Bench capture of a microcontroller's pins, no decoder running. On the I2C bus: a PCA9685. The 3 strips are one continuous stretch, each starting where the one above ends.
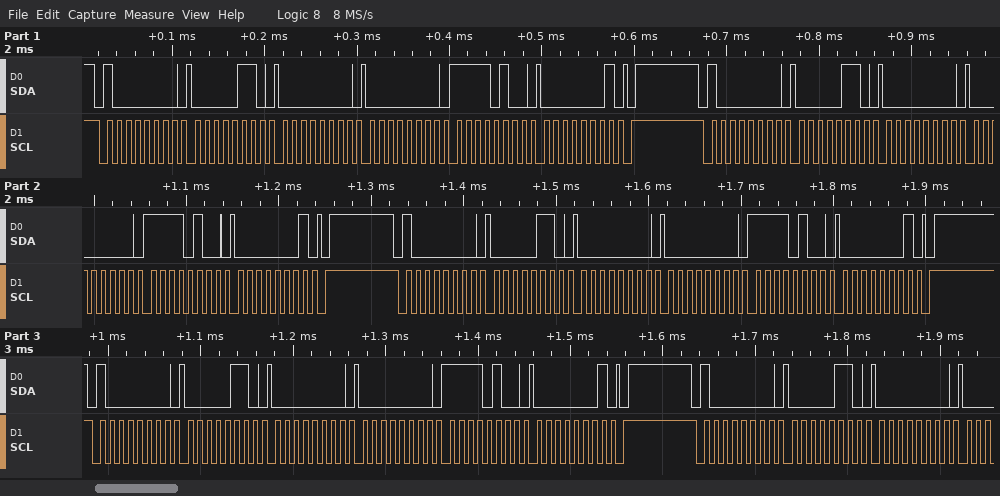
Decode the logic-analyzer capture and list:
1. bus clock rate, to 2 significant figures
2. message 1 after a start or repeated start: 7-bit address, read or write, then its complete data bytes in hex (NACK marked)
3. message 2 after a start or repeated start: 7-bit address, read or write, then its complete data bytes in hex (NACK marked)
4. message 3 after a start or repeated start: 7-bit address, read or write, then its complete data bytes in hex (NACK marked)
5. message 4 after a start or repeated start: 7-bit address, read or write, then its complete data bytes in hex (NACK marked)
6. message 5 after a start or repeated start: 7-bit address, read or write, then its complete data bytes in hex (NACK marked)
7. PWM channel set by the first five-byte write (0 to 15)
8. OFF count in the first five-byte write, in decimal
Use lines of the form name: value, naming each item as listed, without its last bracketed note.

bus clock rate, to 2 significant figures: 100 kHz
message 1 after a start or repeated start: 7-bit address, read or write, then its complete data bytes in hex: 0x40 write: 06 00 00 F4 01
message 2 after a start or repeated start: 7-bit address, read or write, then its complete data bytes in hex: 0x40 write: 06 00 00 F4 01
message 3 after a start or repeated start: 7-bit address, read or write, then its complete data bytes in hex: 0x40 write: 06 00 00 F4 01
message 4 after a start or repeated start: 7-bit address, read or write, then its complete data bytes in hex: 0x40 write: 06 00 00 F4 01
message 5 after a start or repeated start: 7-bit address, read or write, then its complete data bytes in hex: 0x40 write: 06 00
PWM channel set by the first five-byte write: 0
OFF count in the first five-byte write, in decimal: 500
